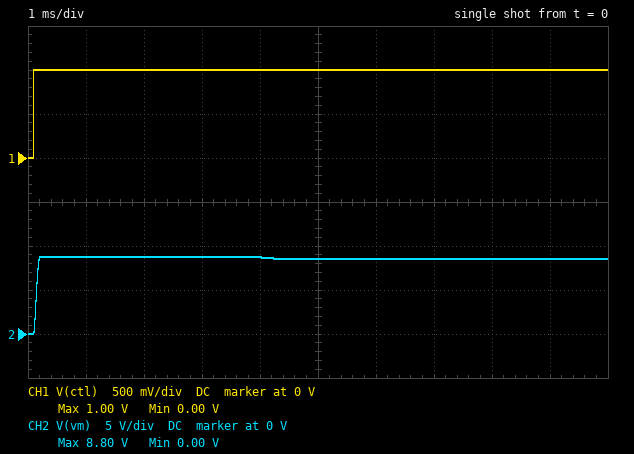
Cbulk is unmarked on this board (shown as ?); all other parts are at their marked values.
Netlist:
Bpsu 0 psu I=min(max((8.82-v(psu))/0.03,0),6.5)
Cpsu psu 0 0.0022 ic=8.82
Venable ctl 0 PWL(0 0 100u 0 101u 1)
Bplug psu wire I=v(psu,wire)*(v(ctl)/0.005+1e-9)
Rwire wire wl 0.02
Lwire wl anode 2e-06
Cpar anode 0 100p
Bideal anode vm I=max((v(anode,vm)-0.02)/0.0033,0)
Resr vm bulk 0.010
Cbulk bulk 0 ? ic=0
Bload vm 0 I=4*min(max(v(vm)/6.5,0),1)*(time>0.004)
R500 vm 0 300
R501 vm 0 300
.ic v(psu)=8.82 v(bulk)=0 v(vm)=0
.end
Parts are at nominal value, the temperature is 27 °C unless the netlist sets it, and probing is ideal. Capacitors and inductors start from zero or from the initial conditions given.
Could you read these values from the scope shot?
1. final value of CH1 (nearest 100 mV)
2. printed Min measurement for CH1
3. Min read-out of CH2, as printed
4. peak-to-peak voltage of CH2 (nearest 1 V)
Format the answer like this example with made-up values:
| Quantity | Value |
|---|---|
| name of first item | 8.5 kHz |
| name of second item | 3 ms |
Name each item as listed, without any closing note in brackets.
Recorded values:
| Quantity | Value |
|---|---|
| final value of CH1 | 1.0 V |
| printed Min measurement for CH1 | 0.00 V |
| Min read-out of CH2, as printed | 0.00 V |
| peak-to-peak voltage of CH2 | 9 V |
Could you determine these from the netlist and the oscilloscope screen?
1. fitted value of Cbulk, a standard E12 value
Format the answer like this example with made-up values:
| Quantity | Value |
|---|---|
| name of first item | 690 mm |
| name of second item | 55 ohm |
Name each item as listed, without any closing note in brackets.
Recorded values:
| Quantity | Value |
|---|---|
| fitted value of Cbulk, a standard E12 value | 820 µF |
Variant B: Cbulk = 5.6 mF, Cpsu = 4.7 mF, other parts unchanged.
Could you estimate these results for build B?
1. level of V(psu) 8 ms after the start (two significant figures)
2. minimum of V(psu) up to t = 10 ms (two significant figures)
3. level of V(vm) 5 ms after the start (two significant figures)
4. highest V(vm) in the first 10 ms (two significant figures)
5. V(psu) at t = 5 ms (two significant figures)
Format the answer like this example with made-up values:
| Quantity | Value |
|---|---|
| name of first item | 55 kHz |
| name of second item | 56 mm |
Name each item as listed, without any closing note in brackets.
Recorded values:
| Quantity | Value |
|---|---|
| level of V(psu) 8 ms after the start | 7.5 V |
| minimum of V(psu) up to t = 10 ms | 4.0 V |
| level of V(vm) 5 ms after the start | 6.6 V |
| highest V(vm) in the first 10 ms | 7.8 V |
| V(psu) at t = 5 ms | 6.8 V |
